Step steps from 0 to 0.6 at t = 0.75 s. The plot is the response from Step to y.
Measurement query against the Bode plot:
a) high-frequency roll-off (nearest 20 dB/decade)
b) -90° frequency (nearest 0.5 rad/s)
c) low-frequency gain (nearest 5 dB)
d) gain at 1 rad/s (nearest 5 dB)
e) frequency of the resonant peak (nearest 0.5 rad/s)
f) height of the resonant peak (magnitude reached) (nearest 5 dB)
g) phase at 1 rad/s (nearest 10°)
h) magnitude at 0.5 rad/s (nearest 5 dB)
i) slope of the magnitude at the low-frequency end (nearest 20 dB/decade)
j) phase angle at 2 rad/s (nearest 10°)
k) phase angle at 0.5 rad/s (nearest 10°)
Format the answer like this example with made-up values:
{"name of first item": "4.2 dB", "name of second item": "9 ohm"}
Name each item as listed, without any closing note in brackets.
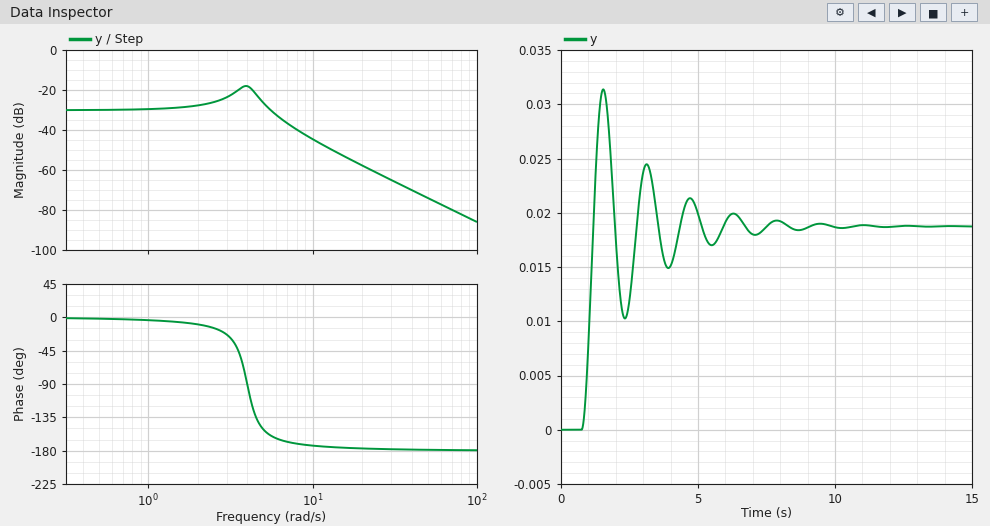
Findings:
{"high-frequency roll-off": "-40 dB/decade", "-90° frequency": "4.0 rad/s", "low-frequency gain": "-30 dB", "gain at 1 rad/s": "-30 dB", "frequency of the resonant peak": "4.0 rad/s", "height of the resonant peak (magnitude reached)": "-20 dB", "phase at 1 rad/s": "0°", "magnitude at 0.5 rad/s": "-30 dB", "slope of the magnitude at the low-frequency end": "0 dB/decade", "phase angle at 2 rad/s": "-10°", "phase angle at 0.5 rad/s": "0°"}
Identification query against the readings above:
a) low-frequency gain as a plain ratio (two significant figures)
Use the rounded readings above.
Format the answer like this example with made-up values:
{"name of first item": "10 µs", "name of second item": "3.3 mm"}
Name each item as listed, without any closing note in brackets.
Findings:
{"low-frequency gain as a plain ratio": "0.032"}
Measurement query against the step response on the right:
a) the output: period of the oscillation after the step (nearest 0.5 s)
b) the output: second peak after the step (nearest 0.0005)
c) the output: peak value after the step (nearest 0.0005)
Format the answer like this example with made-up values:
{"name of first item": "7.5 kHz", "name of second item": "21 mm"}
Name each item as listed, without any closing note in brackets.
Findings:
{"the output: period of the oscillation after the step": "1.5 s", "the output: second peak after the step": "0.0245", "the output: peak value after the step": "0.0315"}
